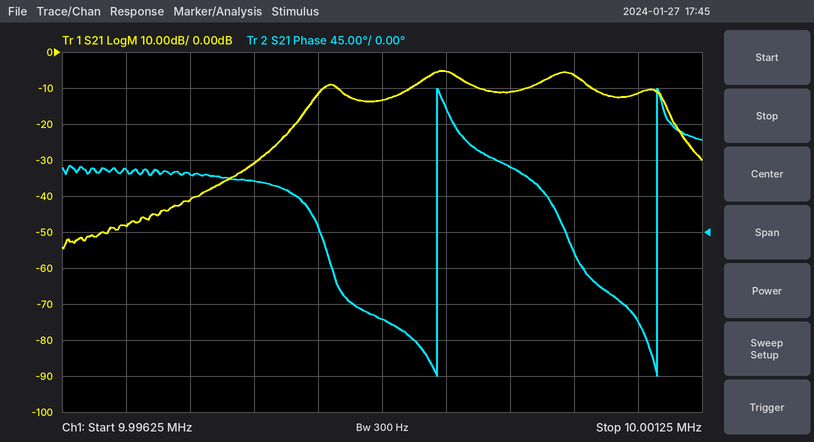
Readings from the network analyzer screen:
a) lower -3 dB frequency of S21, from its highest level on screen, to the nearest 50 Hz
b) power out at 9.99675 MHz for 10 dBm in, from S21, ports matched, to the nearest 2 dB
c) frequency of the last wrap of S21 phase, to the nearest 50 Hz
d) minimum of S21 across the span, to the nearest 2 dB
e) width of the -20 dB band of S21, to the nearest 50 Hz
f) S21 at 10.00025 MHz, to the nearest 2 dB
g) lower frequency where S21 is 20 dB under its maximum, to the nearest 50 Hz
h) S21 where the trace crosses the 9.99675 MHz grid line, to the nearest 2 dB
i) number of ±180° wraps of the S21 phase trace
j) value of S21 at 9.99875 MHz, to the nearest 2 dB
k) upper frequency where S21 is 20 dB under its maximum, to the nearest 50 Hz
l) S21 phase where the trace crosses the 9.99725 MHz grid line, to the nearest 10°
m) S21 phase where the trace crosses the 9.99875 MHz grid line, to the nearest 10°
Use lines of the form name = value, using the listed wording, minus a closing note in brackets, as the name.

lower -3 dB frequency of S21, from its highest level on screen, to the nearest 50 Hz = 9.99905 MHz
power out at 9.99675 MHz for 10 dBm in, from S21, ports matched, to the nearest 2 dB = -38 dBm
frequency of the last wrap of S21 phase, to the nearest 50 Hz = 10.00090 MHz
minimum of S21 across the span, to the nearest 2 dB = -54 dB
width of the -20 dB band of S21, to the nearest 50 Hz = 3.20 kHz
S21 at 10.00025 MHz, to the nearest 2 dB = -6 dB
lower frequency where S21 is 20 dB under its maximum, to the nearest 50 Hz = 9.99795 MHz
S21 where the trace crosses the 9.99675 MHz grid line, to the nearest 2 dB = -48 dB
number of ±180° wraps of the S21 phase trace = 2
value of S21 at 9.99875 MHz, to the nearest 2 dB = -14 dB
upper frequency where S21 is 20 dB under its maximum, to the nearest 50 Hz = 10.00115 MHz
S21 phase where the trace crosses the 9.99725 MHz grid line, to the nearest 10° = 70°
S21 phase where the trace crosses the 9.99875 MHz grid line, to the nearest 10° = -110°
